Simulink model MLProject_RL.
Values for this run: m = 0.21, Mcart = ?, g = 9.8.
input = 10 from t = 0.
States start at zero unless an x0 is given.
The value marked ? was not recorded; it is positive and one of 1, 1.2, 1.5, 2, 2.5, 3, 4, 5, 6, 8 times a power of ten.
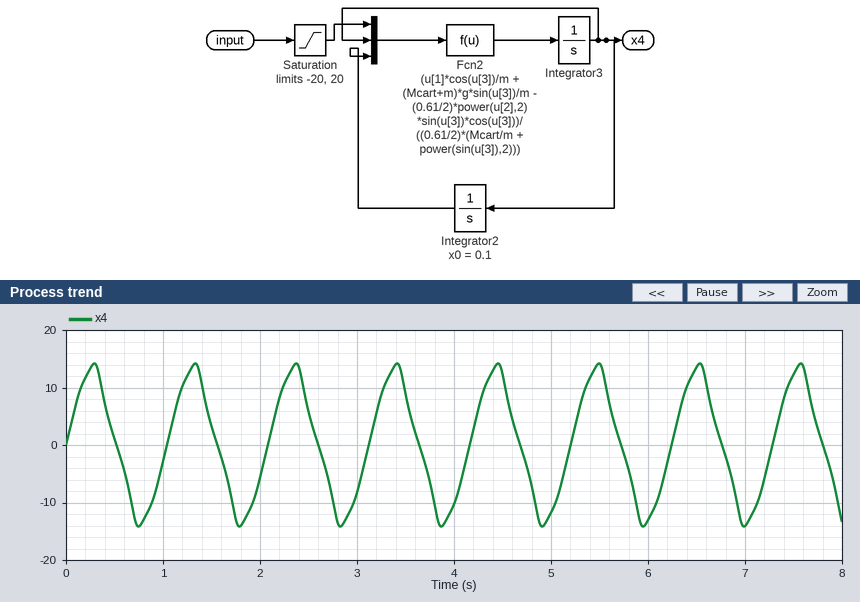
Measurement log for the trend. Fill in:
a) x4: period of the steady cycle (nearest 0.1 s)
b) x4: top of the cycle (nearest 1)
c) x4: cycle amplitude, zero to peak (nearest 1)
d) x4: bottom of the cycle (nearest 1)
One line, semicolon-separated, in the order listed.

1.0 s; 14; 14; -14
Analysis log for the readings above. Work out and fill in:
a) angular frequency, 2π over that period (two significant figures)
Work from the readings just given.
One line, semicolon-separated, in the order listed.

6.3 rad/s
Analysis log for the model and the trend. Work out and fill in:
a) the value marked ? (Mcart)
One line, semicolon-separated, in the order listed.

0.5
